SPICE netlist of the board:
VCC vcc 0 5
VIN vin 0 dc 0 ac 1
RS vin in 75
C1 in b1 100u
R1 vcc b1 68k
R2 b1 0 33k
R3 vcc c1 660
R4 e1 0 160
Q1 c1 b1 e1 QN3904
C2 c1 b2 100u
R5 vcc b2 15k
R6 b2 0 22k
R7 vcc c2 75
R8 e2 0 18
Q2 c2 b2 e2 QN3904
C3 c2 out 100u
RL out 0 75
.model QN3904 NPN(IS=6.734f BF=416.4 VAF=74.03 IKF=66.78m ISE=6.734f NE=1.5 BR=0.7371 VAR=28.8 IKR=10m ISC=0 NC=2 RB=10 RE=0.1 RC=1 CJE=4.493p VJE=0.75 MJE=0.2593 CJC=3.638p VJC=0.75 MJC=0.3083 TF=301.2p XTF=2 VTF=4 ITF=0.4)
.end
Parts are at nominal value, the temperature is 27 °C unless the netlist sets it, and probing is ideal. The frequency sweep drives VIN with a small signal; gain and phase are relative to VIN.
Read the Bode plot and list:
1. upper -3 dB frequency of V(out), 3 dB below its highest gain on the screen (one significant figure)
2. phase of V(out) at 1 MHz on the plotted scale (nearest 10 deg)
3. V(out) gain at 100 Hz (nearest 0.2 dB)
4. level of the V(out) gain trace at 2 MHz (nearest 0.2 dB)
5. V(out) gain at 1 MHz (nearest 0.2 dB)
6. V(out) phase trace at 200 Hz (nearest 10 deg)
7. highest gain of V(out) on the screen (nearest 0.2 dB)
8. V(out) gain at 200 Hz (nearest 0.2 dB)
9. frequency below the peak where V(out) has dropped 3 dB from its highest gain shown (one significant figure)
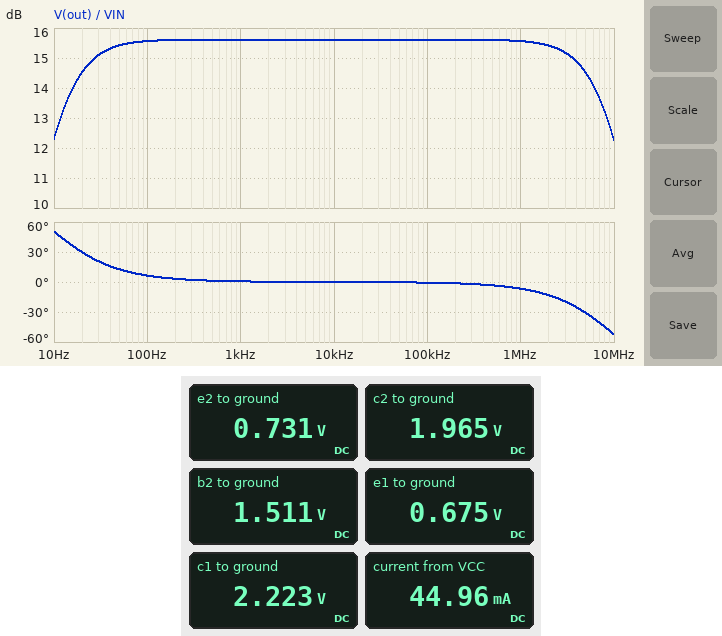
9 MHz
-10 deg
15.6 dB
15.4 dB
15.6 dB
0 deg
15.6 dB
15.6 dB
10 Hz
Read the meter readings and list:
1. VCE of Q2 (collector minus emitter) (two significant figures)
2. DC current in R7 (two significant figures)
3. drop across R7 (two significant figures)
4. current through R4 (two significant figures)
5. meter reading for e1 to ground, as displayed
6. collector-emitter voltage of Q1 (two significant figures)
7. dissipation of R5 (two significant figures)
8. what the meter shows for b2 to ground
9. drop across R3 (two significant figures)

1.2 V
40 mA
3.0 V
4.2 mA
0.675 V
1.5 V
810 µW
1.511 V
2.8 V
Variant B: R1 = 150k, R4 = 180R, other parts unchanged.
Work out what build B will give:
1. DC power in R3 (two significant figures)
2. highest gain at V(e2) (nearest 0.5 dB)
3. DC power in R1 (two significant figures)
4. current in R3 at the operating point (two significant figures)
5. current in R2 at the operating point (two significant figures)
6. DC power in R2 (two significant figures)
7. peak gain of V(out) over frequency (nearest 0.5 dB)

600 µW
7.5 dB
120 µW
950 µA
25 µA
21 µW
13.5 dB
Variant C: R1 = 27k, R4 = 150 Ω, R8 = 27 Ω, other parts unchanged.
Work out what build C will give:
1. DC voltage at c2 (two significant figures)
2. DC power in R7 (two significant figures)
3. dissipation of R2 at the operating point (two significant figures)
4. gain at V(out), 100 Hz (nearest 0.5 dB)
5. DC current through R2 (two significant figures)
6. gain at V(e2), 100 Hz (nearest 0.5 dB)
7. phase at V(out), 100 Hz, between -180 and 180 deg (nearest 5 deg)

2.3 V
96 mW
80 µW
-0.5 dB
49 µA
-3.5 dB
10 deg
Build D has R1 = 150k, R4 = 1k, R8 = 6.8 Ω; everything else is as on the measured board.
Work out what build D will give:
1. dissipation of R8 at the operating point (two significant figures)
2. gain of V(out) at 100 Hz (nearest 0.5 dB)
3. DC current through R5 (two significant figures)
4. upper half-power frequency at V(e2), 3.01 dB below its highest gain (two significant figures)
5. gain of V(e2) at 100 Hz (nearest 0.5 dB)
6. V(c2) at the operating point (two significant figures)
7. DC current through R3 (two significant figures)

16 mW
5.0 dB
260 µA
5.5 MHz
-10.0 dB
1.4 V
250 µA
